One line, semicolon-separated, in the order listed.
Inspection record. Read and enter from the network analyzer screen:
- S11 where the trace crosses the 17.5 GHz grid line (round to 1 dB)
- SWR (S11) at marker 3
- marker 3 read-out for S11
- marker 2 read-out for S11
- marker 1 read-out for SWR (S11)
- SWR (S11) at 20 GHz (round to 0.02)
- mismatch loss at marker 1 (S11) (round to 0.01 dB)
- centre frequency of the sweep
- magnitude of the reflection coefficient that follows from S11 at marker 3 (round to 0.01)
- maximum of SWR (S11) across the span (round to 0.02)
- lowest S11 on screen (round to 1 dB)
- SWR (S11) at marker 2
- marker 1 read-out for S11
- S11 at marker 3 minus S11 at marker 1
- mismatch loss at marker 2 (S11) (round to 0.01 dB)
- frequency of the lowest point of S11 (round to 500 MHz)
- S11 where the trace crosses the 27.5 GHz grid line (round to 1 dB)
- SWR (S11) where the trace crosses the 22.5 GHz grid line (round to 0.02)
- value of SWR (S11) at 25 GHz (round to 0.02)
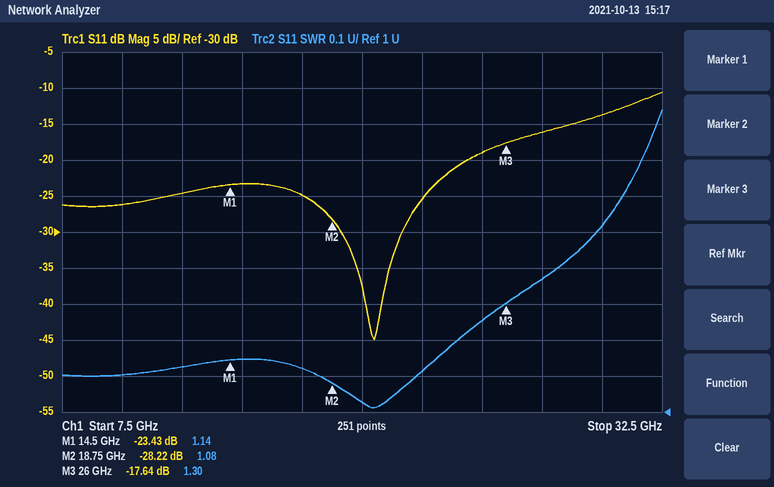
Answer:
-25 dB; 1.30; -17.64 dB; -28.22 dB; 1.14; 1.02; 0.02 dB; 20 GHz; 0.13; 1.84; -45 dB; 1.08; -23.43 dB; 5.79 dB; 0.01 dB; 20.5 GHz; -16 dB; 1.12; 1.26
